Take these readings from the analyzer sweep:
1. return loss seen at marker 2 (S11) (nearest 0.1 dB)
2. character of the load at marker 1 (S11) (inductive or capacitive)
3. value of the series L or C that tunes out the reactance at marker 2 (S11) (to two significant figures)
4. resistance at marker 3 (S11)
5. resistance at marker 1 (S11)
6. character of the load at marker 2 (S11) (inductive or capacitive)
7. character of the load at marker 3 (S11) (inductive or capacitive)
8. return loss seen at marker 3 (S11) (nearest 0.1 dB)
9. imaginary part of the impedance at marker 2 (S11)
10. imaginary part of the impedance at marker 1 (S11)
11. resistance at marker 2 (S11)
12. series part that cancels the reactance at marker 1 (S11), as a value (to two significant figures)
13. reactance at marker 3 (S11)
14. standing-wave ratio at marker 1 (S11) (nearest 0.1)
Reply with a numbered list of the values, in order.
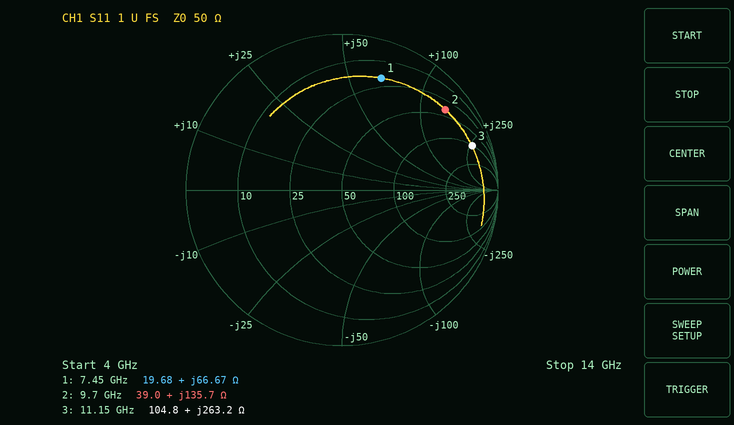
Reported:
1. 1.5 dB
2. inductive
3. 120 fF
4. 104.8 Ω
5. 19.68 Ω
6. inductive
7. inductive
8. 1.1 dB
9. +135.7 Ω
10. +66.67 Ω
11. 39.0 Ω
12. 320 fF
13. +263.2 Ω
14. 7.3
